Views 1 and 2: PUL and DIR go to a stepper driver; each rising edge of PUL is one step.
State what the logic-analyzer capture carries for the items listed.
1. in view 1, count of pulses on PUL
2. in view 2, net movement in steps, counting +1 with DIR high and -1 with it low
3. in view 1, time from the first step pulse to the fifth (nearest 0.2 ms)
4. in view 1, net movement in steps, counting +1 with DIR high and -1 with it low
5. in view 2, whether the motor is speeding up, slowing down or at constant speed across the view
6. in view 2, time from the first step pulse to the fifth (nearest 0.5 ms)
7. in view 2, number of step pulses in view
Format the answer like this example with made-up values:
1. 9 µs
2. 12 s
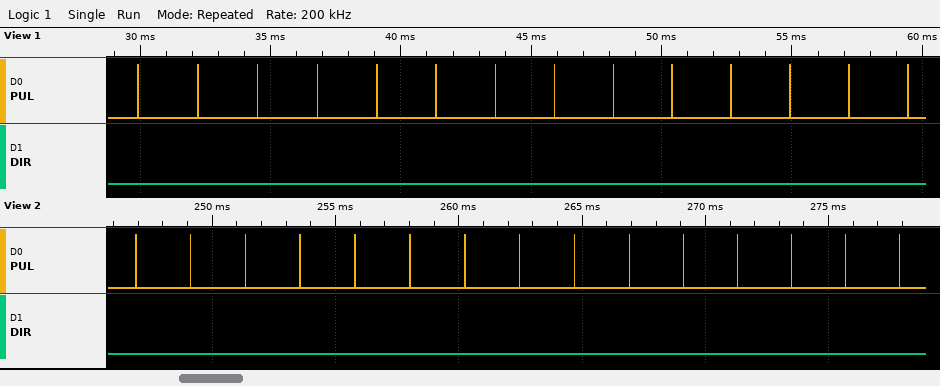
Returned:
1. 14
2. -15
3. 9.2 ms
4. -14
5. constant speed
6. 9.0 ms
7. 15
